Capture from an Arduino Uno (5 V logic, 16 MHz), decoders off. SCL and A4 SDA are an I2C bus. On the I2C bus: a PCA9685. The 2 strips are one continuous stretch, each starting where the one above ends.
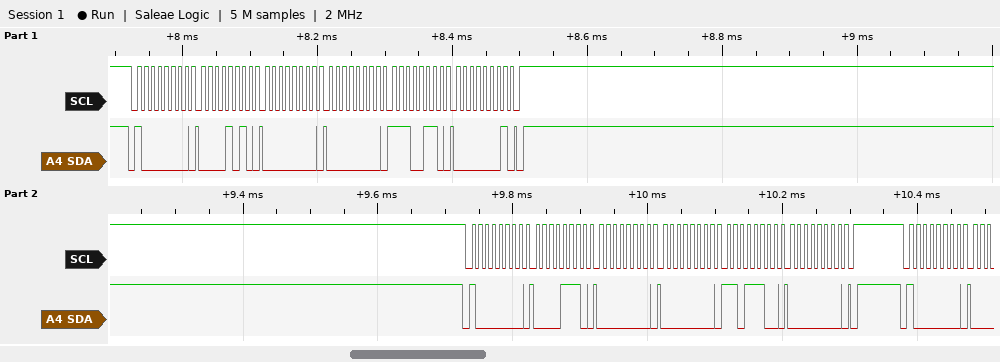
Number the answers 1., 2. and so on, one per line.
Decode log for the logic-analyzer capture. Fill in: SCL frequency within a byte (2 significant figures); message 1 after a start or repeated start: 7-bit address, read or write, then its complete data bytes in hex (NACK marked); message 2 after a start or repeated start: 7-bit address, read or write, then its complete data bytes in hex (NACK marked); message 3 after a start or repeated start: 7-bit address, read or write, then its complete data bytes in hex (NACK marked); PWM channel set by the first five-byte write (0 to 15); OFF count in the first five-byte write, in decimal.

1. 100 kHz
2. 0x40 write: 0A 00 00 E6 01
3. 0x40 write: 0E 00 00 DC 00
4. 0x40 write
5. 1
6. 486
